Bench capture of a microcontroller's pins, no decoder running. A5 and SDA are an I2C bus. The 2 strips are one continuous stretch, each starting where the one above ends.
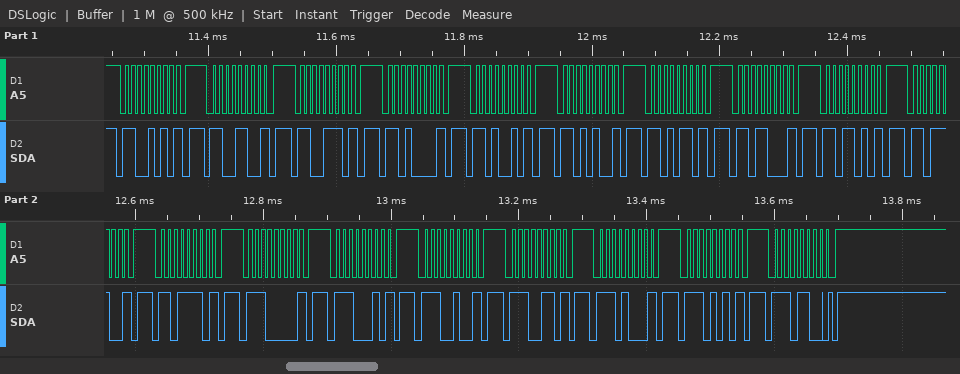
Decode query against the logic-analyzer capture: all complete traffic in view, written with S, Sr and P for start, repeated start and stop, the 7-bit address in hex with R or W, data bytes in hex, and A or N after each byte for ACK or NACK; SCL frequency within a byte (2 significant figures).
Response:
S 65W N P S 66W N P S 67W N P S 68W N P S 69W N P S 6AW N P S 6BW N P S 6CW N P S 6DW N P S 6EW N P S 6FW N P S 70W N P S 71W N P S 72W N P S 73W N P S 74W N P S 75W N P S 76W A P
100 kHz
